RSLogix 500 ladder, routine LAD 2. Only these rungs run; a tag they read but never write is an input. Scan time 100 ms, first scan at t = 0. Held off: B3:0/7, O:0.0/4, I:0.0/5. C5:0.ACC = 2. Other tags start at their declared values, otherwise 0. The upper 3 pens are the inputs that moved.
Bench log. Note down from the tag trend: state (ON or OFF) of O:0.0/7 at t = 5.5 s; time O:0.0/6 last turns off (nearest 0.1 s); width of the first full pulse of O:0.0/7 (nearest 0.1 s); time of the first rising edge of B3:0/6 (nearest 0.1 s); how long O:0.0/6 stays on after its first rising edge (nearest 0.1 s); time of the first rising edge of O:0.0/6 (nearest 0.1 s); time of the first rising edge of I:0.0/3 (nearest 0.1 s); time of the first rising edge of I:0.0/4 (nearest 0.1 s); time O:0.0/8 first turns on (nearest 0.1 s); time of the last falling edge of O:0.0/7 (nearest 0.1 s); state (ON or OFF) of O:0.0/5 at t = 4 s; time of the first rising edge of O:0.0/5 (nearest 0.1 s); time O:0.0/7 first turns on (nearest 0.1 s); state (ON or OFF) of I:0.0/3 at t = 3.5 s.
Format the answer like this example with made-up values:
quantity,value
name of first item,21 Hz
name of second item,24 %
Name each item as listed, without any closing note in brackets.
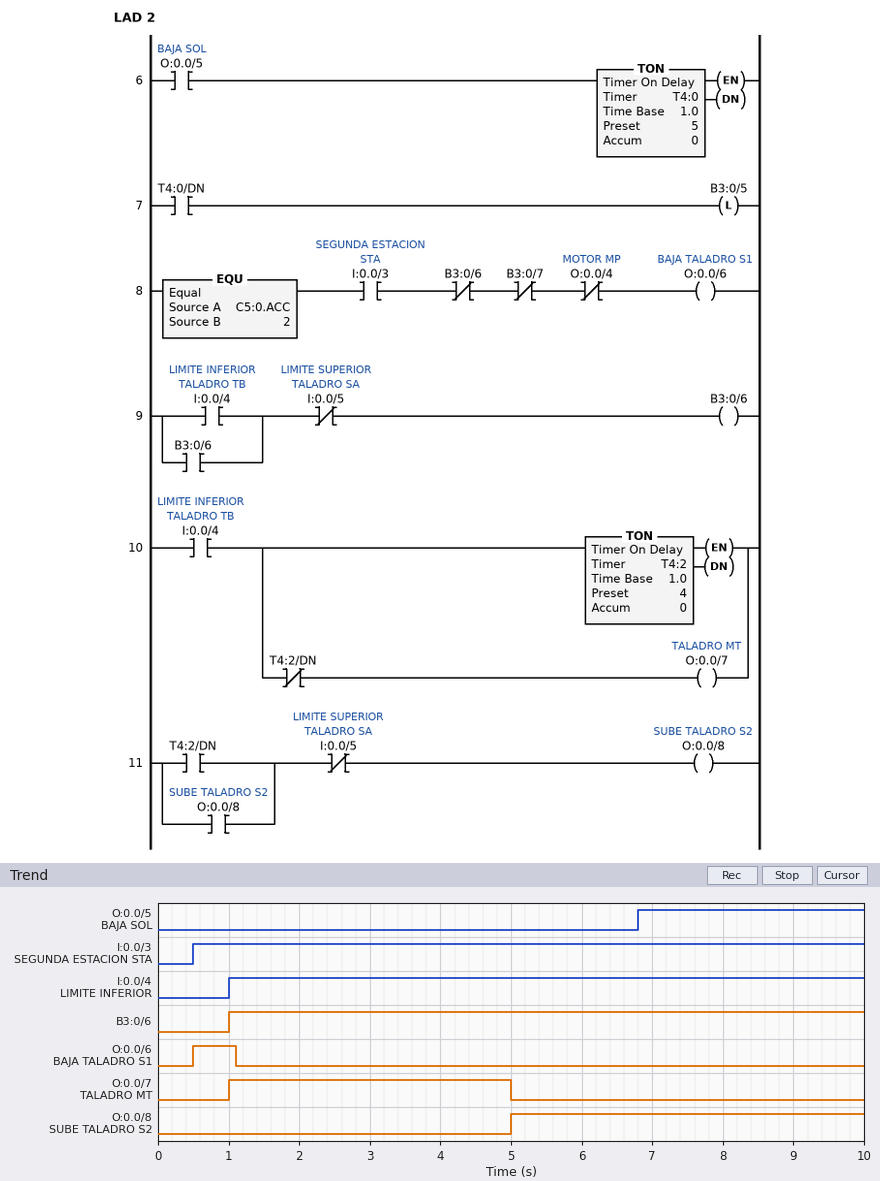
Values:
quantity,value
state (ON or OFF) of O:0.0/7 at t = 5.5 s,OFF
time O:0.0/6 last turns off,1.1 s
width of the first full pulse of O:0.0/7,4.0 s
time of the first rising edge of B3:0/6,1.0 s
how long O:0.0/6 stays on after its first rising edge,0.6 s
time of the first rising edge of O:0.0/6,0.5 s
time of the first rising edge of I:0.0/3,0.5 s
time of the first rising edge of I:0.0/4,1.0 s
time O:0.0/8 first turns on,5.0 s
time of the last falling edge of O:0.0/7,5.0 s
state (ON or OFF) of O:0.0/5 at t = 4 s,OFF
time of the first rising edge of O:0.0/5,6.8 s
time O:0.0/7 first turns on,1.0 s
state (ON or OFF) of I:0.0/3 at t = 3.5 s,ON
